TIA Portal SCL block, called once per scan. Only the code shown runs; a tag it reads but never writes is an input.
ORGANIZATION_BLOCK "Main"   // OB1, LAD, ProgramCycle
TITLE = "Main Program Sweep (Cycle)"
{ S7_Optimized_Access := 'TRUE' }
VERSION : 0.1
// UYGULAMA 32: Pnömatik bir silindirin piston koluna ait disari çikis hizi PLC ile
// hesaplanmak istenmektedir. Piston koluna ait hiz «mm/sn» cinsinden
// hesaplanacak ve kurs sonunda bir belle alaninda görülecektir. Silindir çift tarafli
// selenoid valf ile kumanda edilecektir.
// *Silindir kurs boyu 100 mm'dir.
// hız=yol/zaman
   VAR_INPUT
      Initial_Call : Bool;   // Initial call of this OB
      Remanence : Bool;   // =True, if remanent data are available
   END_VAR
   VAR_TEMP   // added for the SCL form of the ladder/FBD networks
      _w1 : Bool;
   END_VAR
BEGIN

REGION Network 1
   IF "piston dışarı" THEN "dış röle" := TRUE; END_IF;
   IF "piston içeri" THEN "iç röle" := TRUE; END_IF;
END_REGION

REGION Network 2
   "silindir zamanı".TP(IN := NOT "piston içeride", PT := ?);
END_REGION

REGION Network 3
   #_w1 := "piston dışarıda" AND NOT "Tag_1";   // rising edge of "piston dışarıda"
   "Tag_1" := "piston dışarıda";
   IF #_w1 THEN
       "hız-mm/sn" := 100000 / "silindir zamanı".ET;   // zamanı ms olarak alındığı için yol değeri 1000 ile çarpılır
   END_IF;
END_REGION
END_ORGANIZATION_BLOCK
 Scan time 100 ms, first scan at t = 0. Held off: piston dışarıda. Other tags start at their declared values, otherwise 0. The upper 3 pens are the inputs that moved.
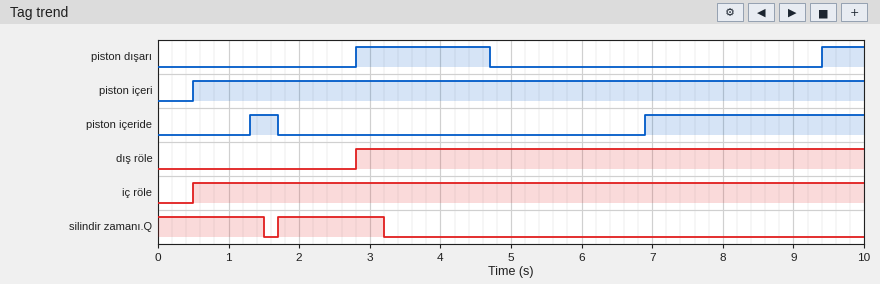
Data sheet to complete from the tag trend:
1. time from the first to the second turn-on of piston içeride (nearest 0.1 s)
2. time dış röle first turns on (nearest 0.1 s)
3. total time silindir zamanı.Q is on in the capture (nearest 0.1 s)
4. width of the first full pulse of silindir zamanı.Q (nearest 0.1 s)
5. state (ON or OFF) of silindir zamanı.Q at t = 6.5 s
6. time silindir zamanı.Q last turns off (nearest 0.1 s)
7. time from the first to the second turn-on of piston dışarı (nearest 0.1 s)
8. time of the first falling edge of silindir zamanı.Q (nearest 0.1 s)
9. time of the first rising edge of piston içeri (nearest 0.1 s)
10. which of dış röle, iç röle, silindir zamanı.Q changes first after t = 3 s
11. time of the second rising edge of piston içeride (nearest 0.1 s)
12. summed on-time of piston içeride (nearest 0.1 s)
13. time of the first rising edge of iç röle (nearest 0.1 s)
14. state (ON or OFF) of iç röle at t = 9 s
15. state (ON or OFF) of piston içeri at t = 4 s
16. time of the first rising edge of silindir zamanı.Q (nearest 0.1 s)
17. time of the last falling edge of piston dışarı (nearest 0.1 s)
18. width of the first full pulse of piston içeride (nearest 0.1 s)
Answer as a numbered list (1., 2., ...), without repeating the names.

1. 5.6 s
2. 2.8 s
3. 3.0 s
4. 1.5 s
5. OFF
6. 3.2 s
7. 6.6 s
8. 1.5 s
9. 0.5 s
10. silindir zamanı.Q
11. 6.9 s
12. 3.5 s
13. 0.5 s
14. ON
15. ON
16. 1.7 s
17. 4.7 s
18. 0.4 s
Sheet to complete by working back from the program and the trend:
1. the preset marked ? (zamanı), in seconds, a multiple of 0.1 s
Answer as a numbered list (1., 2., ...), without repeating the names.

1. 1.5 s
